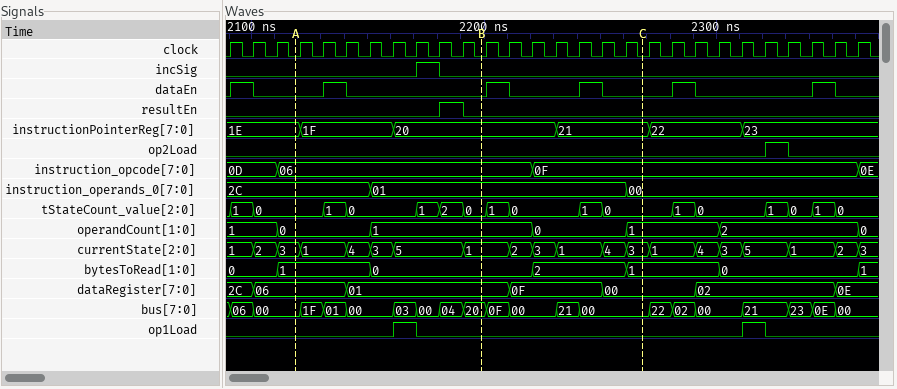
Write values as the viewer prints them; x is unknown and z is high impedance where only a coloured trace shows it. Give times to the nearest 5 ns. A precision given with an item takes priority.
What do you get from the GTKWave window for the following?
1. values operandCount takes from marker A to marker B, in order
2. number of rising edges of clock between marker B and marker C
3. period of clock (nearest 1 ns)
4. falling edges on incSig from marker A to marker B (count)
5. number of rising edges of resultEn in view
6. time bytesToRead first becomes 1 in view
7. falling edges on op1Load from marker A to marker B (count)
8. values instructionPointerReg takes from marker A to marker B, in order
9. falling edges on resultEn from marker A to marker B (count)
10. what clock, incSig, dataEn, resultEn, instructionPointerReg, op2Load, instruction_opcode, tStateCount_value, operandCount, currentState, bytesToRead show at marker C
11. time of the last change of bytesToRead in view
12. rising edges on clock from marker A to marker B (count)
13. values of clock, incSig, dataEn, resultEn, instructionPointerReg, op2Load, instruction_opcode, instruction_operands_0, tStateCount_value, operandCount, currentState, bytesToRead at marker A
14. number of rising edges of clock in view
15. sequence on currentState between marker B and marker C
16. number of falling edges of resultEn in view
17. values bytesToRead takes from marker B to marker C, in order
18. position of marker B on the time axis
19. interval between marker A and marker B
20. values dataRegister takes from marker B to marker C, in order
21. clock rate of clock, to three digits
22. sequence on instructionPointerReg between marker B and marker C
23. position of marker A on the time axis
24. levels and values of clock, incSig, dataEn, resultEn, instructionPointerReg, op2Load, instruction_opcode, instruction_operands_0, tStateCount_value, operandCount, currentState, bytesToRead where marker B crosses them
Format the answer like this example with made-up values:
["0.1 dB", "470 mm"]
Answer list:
["0, 1", "7", "10 ns", "1", "1", "2110 ns", "1", "1E, 1F, 20", "1", "clock=0, incSig=0, dataEn=0, resultEn=0, instructionPointerReg=21, op2Load=0, instruction_opcode=0F, tStateCount_value=0, operandCount=1, currentState=3, bytesToRead=1", "2360 ns", "8", "clock=0, incSig=0, dataEn=0, resultEn=0, instructionPointerReg=1E, op2Load=0, instruction_opcode=06, instruction_operands_0=2C, tStateCount_value=0, operandCount=0, currentState=3, bytesToRead=1", "28", "1, 2, 3, 1, 4, 3", "1", "0, 2, 1", "2200 ns", "80 ns", "01, 0F, 00", "100 MHz", "20, 21", "2120 ns", "clock=0, incSig=0, dataEn=0, resultEn=0, instructionPointerReg=20, op2Load=0, instruction_opcode=06, instruction_operands_0=01, tStateCount_value=0, operandCount=1, currentState=1, bytesToRead=0"]
